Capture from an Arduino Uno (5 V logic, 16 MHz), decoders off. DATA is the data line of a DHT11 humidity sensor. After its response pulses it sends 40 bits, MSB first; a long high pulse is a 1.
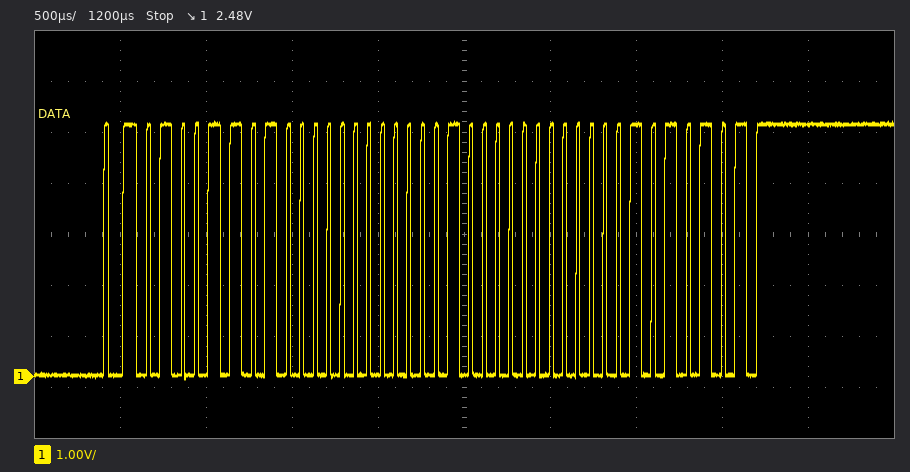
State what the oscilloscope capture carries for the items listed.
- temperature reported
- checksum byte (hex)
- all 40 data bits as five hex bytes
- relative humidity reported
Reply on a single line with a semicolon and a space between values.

8.0 °C; 0x55; 4D 00 08 00 55; 77 %
